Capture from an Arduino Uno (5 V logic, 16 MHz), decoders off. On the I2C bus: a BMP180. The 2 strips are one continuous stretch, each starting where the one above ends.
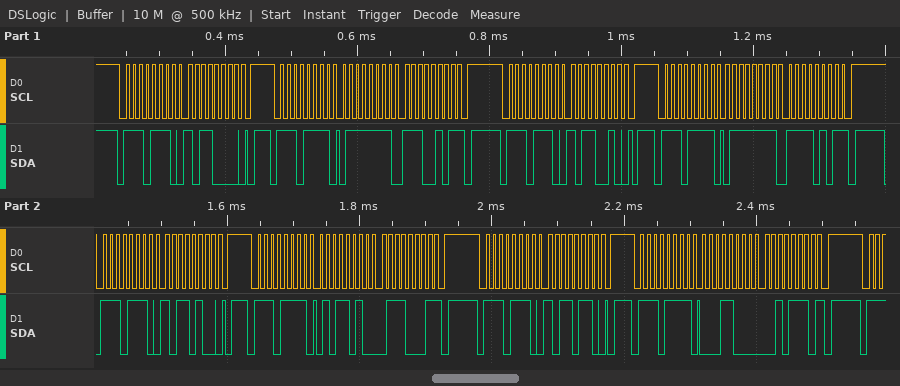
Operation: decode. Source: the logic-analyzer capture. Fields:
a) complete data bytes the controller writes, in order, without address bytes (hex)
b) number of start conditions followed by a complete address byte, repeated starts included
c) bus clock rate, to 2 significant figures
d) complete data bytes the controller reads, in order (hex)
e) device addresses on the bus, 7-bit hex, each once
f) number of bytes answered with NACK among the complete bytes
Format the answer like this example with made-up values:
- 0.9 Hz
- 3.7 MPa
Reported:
- B0 B2 B4 B6
- 8
- 100 kHz
- 7F E5 7F F5 5A 71 18 2E
- 0x77
- 4
